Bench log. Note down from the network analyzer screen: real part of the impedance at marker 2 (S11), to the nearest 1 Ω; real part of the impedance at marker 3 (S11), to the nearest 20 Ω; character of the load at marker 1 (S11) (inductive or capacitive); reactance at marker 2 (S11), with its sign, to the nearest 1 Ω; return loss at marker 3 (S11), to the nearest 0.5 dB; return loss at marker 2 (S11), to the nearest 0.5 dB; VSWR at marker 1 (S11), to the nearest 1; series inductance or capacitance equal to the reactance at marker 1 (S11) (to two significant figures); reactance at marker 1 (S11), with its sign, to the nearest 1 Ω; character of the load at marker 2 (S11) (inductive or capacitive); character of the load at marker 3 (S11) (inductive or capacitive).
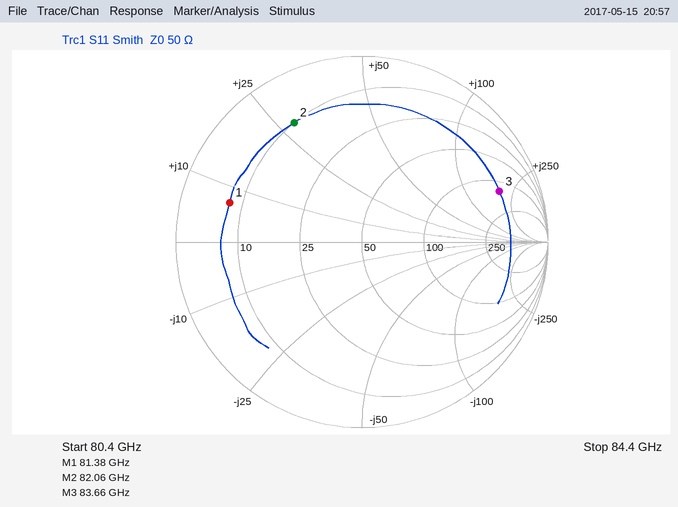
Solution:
10 Ω
140 Ω
inductive
+28 Ω
2.0 dB
2.5 dB
7
14 pH
+7 Ω
inductive
inductive
